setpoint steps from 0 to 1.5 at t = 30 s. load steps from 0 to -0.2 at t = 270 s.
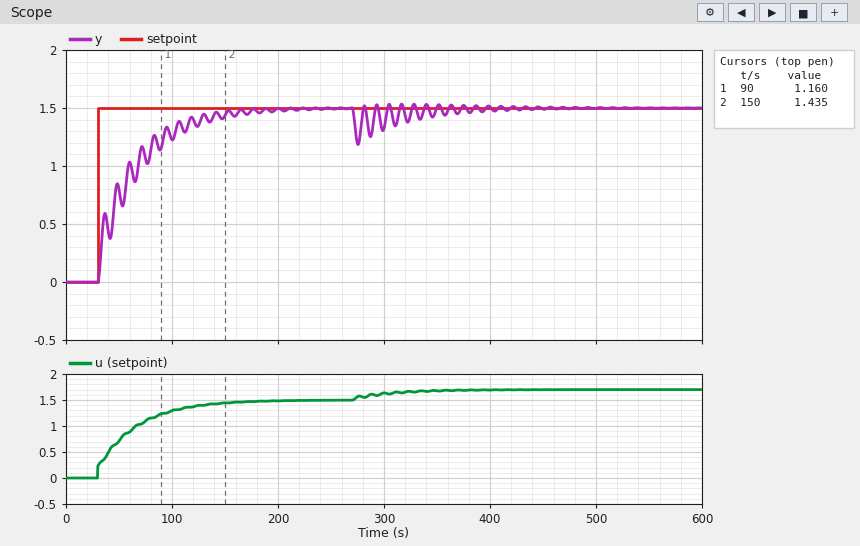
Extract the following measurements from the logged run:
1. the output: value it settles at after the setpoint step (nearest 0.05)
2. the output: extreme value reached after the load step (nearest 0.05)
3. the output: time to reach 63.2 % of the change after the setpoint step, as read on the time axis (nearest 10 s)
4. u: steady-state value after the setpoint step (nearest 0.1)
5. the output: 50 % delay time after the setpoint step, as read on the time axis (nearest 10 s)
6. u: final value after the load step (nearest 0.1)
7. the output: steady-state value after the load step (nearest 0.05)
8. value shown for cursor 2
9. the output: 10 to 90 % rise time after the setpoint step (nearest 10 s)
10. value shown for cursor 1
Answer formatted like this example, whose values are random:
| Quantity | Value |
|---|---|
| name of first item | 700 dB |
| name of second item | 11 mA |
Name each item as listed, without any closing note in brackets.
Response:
| Quantity | Value |
|---|---|
| the output: value it settles at after the setpoint step | 1.50 |
| the output: extreme value reached after the load step | 1.20 |
| the output: time to reach 63.2 % of the change after the setpoint step, as read on the time axis | 60 s |
| u: steady-state value after the setpoint step | 1.5 |
| the output: 50 % delay time after the setpoint step, as read on the time axis | 50 s |
| u: final value after the load step | 1.7 |
| the output: steady-state value after the load step | 1.50 |
| value shown for cursor 2 | 1.435 |
| the output: 10 to 90 % rise time after the setpoint step | 70 s |
| value shown for cursor 1 | 1.160 |
